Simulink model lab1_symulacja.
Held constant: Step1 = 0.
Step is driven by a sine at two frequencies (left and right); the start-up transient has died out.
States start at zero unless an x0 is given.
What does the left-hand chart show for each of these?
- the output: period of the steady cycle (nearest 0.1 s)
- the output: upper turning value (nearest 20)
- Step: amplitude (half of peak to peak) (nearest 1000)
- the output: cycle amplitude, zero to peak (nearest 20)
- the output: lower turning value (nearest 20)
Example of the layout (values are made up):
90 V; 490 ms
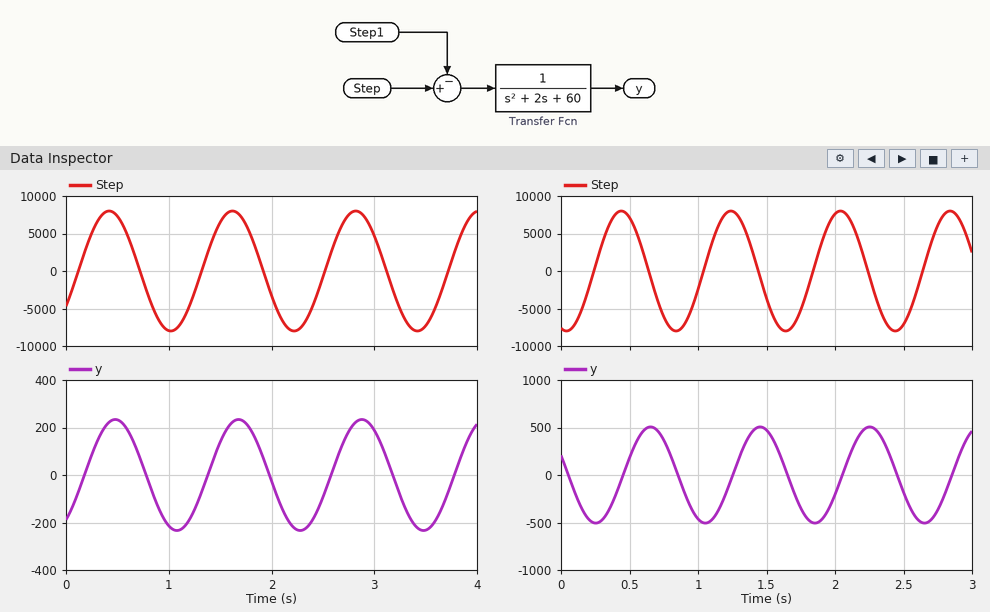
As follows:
1.2 s; 240; 8000; 240; -240
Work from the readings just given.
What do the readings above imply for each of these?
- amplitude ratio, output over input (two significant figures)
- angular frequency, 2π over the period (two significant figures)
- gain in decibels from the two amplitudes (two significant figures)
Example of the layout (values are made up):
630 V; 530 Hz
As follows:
0.030; 5.2 rad/s; -30 dB
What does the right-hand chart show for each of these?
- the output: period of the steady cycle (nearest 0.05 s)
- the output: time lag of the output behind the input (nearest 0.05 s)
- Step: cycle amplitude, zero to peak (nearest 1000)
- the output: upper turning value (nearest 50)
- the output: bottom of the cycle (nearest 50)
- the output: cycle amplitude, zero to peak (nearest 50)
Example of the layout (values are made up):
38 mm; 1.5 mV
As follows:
0.80 s; 0.20 s; 8000; 500; -500; 500
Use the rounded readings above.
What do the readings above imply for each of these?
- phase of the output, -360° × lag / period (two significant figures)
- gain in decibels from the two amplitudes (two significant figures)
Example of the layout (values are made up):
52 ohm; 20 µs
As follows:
-90°; -24 dB
